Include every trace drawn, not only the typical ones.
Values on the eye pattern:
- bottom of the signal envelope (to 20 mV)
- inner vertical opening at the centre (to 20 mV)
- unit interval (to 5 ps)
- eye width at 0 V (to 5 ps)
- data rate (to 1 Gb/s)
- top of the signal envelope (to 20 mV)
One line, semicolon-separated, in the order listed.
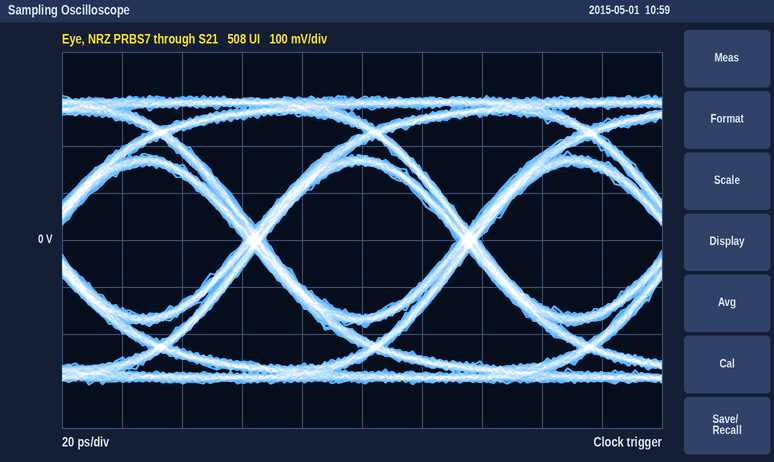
-300 mV; 320 mV; 70 ps; 65 ps; 14 Gb/s; 300 mV
